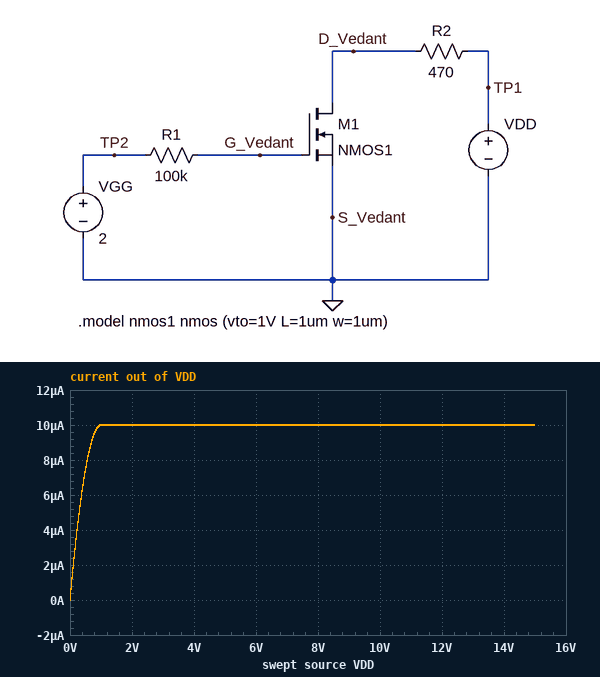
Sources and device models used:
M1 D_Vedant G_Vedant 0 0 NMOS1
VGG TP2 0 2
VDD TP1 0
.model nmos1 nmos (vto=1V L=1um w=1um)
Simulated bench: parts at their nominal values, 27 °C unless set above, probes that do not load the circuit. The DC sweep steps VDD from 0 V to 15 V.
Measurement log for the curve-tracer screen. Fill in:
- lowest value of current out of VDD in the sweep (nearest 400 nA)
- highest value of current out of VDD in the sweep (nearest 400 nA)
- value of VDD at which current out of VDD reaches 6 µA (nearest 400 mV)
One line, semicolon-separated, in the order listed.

0 A; 10.0 µA; 400 mV
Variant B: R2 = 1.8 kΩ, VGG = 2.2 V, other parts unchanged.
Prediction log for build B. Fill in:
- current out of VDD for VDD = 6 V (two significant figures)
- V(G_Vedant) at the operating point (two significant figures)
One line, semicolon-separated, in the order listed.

14 µA; 2.2 V
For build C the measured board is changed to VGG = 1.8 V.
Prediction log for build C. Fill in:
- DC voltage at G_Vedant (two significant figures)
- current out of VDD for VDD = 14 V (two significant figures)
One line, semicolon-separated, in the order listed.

1.8 V; 6.4 µA
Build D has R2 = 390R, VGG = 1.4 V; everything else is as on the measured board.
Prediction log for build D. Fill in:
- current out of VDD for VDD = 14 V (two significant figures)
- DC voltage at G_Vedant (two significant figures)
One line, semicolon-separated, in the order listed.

1.6 µA; 1.4 V
